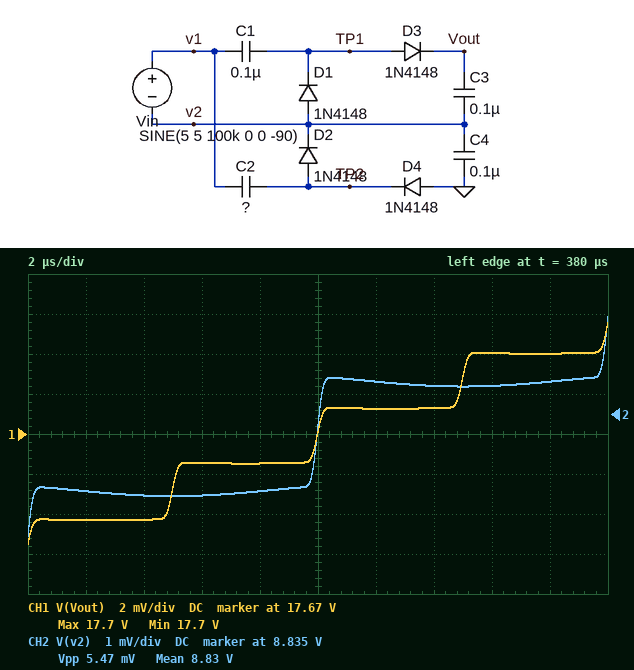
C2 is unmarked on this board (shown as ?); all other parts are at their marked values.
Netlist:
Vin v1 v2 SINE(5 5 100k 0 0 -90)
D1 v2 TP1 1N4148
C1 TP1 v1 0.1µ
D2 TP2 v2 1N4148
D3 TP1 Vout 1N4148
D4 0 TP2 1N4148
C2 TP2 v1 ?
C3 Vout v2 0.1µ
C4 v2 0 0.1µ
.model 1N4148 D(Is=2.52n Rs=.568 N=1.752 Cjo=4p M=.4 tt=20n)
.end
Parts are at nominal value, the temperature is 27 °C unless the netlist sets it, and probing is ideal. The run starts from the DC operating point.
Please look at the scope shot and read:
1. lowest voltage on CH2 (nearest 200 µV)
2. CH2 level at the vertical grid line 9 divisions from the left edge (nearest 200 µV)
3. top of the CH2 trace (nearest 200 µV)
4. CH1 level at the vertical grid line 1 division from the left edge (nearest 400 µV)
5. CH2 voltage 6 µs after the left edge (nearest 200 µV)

8.8320 V
8.8358 V
8.8374 V
17.6696 V
8.8330 V
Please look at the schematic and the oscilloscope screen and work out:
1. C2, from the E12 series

150 nF
